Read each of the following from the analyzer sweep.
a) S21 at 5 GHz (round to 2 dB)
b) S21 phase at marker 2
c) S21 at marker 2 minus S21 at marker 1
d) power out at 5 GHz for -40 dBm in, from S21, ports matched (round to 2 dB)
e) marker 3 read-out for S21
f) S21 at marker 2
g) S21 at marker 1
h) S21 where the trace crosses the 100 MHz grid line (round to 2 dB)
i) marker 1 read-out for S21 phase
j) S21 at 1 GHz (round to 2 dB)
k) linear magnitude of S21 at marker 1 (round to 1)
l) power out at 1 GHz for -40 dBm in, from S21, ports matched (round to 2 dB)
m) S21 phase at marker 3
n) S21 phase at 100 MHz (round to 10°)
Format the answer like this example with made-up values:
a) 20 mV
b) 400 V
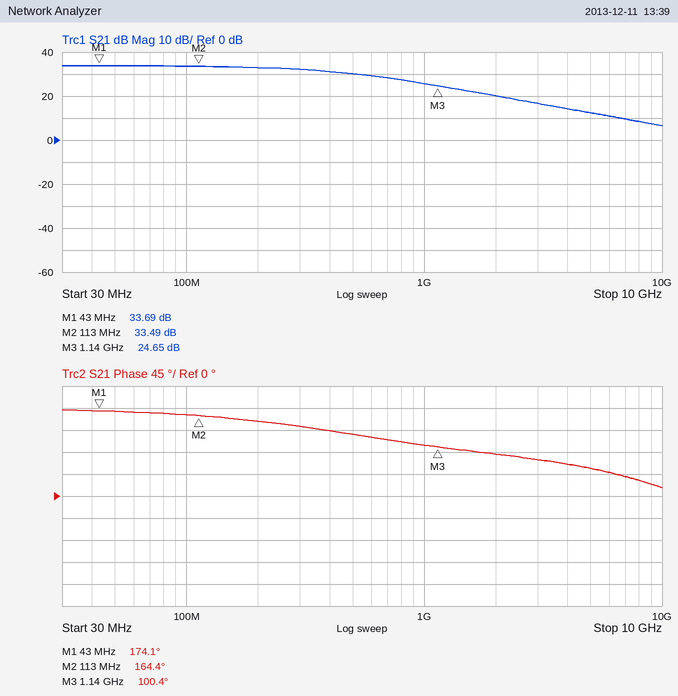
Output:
a) 12 dB
b) 164.4°
c) -0.20 dB
d) -28 dBm
e) 24.65 dB
f) 33.49 dB
g) 33.69 dB
h) 34 dB
i) 174.1°
j) 26 dB
k) 48
l) -14 dBm
m) 100.4°
n) 170°
